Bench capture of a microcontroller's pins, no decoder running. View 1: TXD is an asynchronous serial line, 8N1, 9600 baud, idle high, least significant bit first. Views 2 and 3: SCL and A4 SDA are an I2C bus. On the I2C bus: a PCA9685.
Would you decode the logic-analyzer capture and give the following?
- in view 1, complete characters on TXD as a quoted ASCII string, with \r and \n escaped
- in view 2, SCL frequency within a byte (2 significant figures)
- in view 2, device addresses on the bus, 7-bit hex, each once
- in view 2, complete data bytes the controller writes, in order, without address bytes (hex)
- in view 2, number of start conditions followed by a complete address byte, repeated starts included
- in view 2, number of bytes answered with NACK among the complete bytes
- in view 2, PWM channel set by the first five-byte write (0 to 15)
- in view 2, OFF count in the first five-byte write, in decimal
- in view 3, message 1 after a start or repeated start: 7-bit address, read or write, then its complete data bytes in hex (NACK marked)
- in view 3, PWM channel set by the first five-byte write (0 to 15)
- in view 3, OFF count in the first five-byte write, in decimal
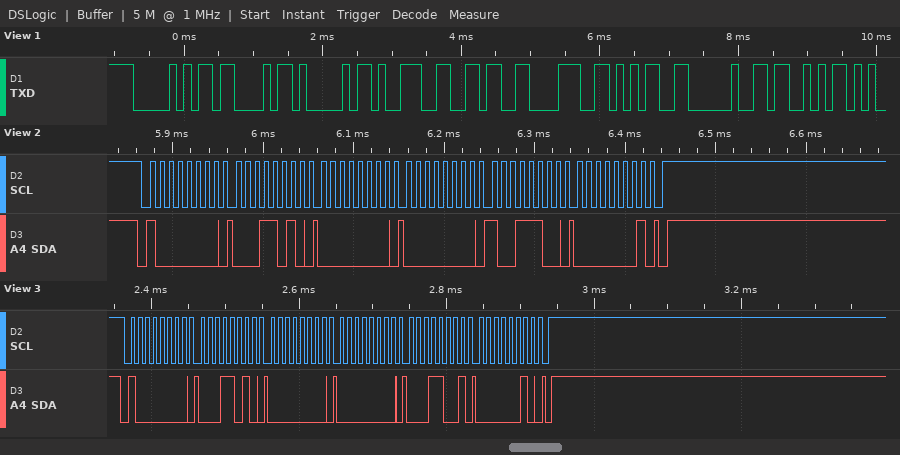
"PCA9685 S"
100 kHz
0x40
1A 00 00 9C 01
1
0
5
412
0x40 write: 1A 00 00 19 02
5
537
